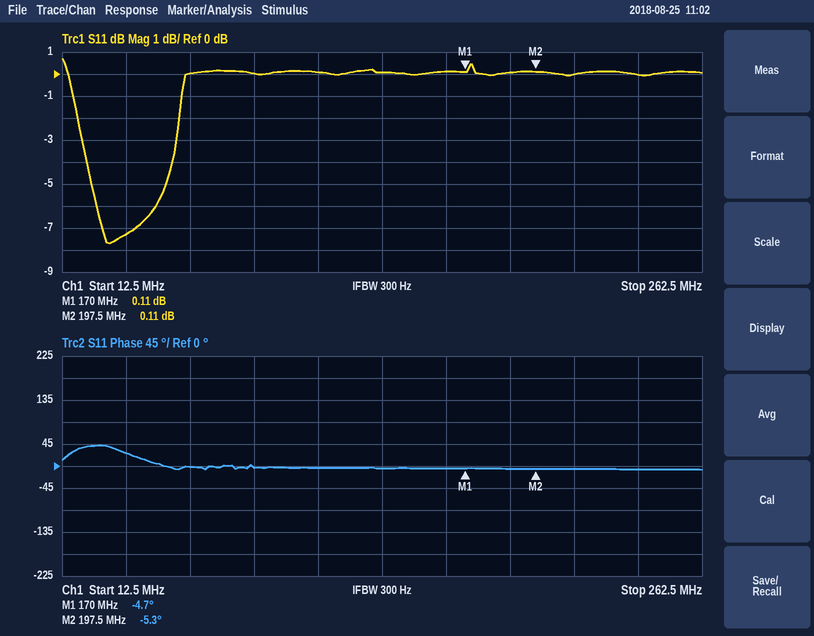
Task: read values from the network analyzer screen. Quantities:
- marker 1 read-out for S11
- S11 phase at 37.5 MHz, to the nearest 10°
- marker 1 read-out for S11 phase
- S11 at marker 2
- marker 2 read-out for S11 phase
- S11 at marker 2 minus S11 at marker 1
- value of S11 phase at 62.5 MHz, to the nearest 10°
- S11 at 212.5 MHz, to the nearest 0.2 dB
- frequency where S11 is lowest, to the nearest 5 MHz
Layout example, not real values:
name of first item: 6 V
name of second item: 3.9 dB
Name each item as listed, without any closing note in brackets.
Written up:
marker 1 read-out for S11: 0.11 dB
S11 phase at 37.5 MHz, to the nearest 10°: 30°
marker 1 read-out for S11 phase: -4.7°
S11 at marker 2: 0.11 dB
marker 2 read-out for S11 phase: -5.3°
S11 at marker 2 minus S11 at marker 1: 0.00 dB
value of S11 phase at 62.5 MHz, to the nearest 10°: 0°
S11 at 212.5 MHz, to the nearest 0.2 dB: 0.0 dB
frequency where S11 is lowest, to the nearest 5 MHz: 30 MHz
